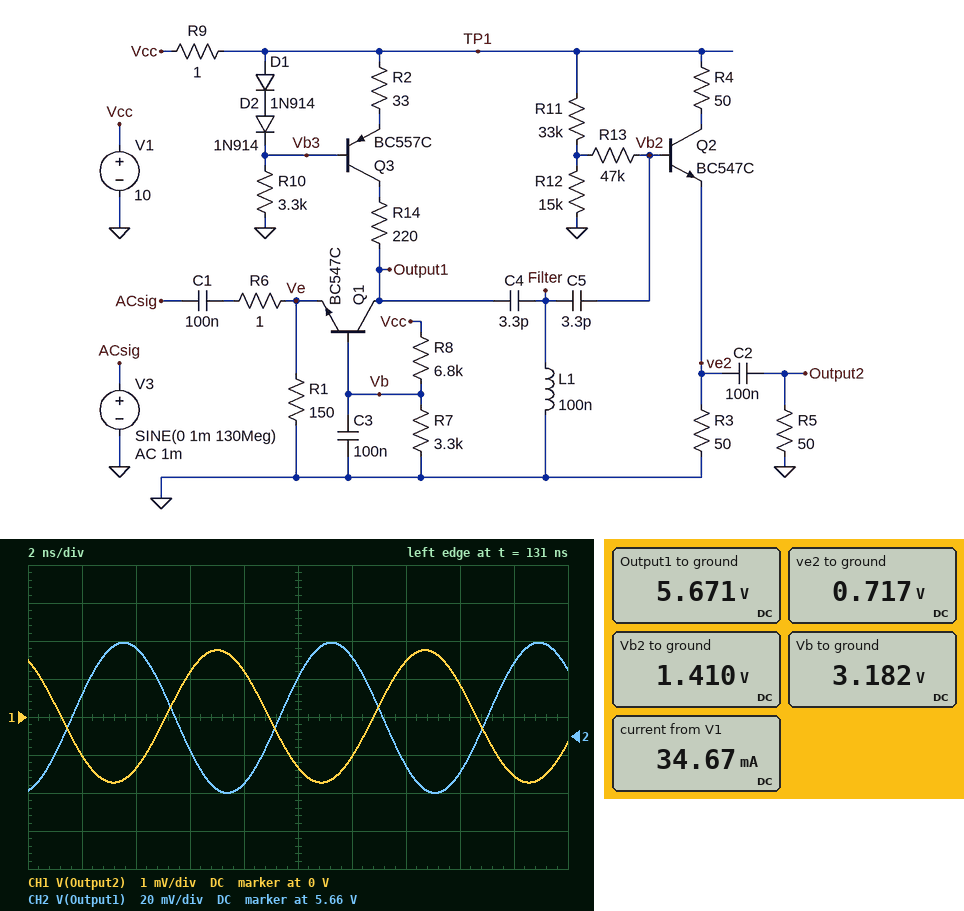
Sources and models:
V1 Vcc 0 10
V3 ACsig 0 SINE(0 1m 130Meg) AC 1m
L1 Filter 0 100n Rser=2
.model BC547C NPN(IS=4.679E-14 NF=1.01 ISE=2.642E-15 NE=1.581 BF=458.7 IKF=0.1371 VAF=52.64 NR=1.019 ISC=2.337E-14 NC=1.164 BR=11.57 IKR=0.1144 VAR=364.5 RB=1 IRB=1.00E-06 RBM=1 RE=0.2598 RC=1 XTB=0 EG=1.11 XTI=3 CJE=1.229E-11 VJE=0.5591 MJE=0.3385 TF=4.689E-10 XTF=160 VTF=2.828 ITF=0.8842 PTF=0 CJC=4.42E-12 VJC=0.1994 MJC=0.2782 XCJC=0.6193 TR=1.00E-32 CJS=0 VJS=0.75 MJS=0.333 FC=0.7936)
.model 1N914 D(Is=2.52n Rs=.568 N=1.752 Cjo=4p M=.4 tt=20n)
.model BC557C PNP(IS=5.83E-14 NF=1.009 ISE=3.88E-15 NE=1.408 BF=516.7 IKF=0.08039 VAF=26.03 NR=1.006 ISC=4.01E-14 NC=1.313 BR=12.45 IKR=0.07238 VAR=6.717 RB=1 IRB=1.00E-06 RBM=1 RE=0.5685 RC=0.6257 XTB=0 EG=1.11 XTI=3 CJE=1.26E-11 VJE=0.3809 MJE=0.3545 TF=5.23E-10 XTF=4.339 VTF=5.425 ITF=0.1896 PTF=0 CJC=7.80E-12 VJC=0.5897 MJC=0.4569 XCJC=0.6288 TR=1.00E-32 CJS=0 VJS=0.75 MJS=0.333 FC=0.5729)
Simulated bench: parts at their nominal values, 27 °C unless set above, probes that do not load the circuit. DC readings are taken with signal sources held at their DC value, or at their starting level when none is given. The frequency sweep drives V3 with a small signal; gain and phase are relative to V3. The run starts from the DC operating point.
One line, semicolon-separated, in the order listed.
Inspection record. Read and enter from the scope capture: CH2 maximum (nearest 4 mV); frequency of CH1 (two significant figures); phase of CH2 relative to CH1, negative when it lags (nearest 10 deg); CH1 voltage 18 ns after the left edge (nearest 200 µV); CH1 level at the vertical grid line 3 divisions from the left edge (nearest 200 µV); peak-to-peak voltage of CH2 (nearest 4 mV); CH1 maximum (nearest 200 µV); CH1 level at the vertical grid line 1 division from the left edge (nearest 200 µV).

5.708 V; 130 MHz; 160 deg; -1.6 mV; 1.2 mV; 80 mV; 1.8 mV; -1.0 mV
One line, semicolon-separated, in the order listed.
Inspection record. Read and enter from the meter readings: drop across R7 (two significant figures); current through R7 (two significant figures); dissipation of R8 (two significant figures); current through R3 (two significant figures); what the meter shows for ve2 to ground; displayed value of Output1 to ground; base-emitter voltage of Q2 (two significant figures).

3.2 V; 960 µA; 6.8 mW; 14 mA; 0.717 V; 5.671 V; 690 mV
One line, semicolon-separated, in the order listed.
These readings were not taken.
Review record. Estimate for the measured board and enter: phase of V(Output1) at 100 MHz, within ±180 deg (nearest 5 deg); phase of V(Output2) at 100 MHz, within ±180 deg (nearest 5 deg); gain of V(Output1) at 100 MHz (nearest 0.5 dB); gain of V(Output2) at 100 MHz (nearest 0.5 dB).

-65 deg; 130 deg; 34.0 dB; -0.5 dB
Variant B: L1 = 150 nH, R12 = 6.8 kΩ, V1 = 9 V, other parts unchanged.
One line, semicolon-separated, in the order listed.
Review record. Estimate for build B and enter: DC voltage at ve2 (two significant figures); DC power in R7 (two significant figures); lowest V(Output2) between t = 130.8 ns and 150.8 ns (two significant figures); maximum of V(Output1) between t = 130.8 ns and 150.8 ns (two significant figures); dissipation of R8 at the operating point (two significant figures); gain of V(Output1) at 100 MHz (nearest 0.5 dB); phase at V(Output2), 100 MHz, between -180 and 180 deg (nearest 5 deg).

280 mV; 2.5 mW; -3.1 mV; 5.3 V; 5.5 mW; 33.5 dB; 140 deg
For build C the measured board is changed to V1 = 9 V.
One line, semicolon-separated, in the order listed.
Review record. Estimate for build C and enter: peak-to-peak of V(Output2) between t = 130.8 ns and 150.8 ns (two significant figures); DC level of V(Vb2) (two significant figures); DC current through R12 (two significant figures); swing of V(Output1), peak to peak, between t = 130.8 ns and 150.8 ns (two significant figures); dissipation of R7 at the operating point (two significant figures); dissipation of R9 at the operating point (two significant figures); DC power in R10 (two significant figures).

3.3 mV; 1.3 V; 170 µA; 77 mV; 2.5 mW; 870 µW; 18 mW
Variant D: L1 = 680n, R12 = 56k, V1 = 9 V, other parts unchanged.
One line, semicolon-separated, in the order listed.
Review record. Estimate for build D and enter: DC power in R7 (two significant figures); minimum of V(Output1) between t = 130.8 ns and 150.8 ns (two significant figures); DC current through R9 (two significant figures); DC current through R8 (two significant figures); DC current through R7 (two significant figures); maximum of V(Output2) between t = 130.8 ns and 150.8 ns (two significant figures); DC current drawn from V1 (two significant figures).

2.5 mW; 5.2 V; 41 mA; 900 µA; 870 µA; 5.1 mV; 42 mA
